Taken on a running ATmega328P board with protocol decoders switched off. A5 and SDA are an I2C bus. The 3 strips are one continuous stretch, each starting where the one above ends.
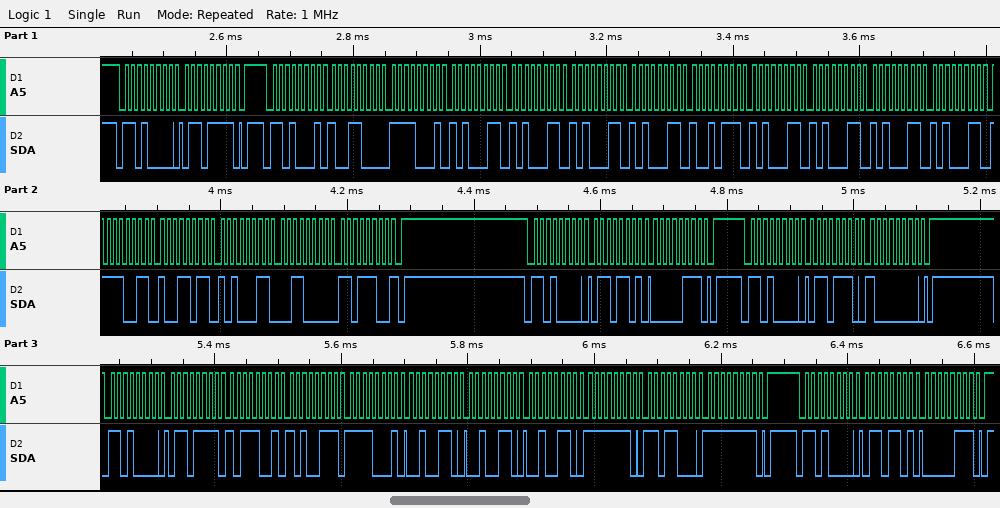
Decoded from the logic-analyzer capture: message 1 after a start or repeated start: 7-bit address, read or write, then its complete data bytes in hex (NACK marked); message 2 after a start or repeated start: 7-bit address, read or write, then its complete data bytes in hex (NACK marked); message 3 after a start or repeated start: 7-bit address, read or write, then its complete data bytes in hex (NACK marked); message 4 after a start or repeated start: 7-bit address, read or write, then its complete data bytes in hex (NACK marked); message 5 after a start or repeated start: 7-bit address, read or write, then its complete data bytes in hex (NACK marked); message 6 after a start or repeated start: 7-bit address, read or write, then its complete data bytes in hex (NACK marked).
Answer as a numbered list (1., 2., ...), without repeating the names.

1. 0x68 write: 6F
2. 0x68 read: 98 F1 A3 A3 A3 A3 97 A3 A3 A3 A3 F3 9B A3 30 DC NACK
3. 0x68 write: 6D 07
4. 0x68 write: 6E 80
5. 0x68 write: 6F B9 A7 F1 26 26 26 FE D8 FF
6. 0x68 write: 6D 07
